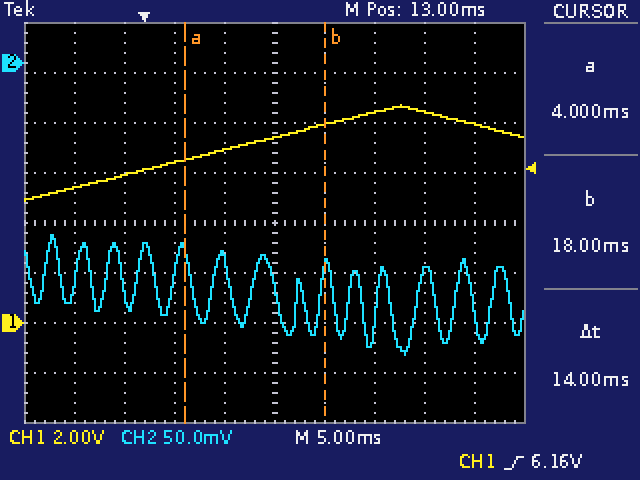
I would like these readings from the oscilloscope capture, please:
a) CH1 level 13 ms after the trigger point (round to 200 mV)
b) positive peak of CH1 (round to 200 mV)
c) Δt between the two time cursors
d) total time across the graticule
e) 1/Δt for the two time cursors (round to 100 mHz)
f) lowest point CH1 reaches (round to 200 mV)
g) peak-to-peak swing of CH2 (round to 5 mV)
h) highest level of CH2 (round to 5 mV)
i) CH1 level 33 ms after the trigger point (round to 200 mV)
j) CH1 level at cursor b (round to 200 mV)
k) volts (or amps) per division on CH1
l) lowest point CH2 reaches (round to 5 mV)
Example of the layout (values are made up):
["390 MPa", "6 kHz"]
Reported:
["7.4 V", "8.8 V", "14 ms", "50 ms", "71.4 Hz", "4.8 V", "120 mV", "-170 mV", "8.0 V", "8.0 V", "2 V", "-290 mV"]
